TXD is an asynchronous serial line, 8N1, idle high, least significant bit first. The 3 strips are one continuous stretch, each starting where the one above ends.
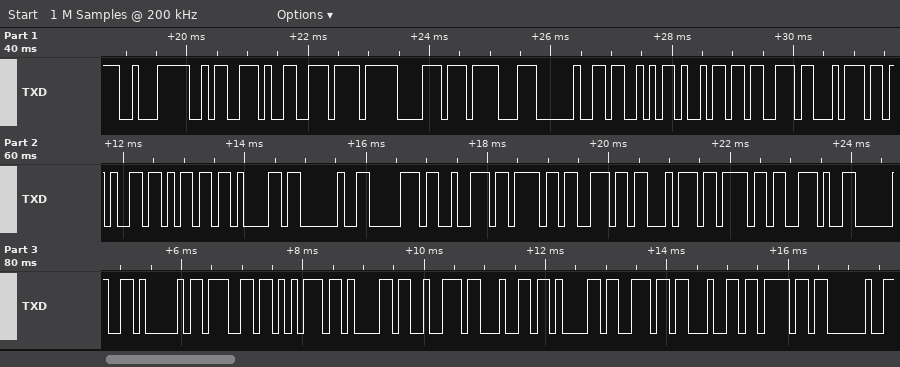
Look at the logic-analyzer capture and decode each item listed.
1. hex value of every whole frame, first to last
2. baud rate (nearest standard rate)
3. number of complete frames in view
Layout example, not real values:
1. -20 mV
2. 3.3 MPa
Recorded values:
1. 0xE2 0x9A 0x99 0xEF 0xB8 0x8F 0x20 0x53 0x69 0x73 0x74 0x65 0x6D 0x61 0x20 0x70 0x72 0x6F 0x6E 0x74 0x6F 0x2E 0x20 0x41 0x67 0x75 0x61 0x72 0x64 0x61 0x6E 0x64 0x6F 0x20
2. 9600 baud
3. 34
